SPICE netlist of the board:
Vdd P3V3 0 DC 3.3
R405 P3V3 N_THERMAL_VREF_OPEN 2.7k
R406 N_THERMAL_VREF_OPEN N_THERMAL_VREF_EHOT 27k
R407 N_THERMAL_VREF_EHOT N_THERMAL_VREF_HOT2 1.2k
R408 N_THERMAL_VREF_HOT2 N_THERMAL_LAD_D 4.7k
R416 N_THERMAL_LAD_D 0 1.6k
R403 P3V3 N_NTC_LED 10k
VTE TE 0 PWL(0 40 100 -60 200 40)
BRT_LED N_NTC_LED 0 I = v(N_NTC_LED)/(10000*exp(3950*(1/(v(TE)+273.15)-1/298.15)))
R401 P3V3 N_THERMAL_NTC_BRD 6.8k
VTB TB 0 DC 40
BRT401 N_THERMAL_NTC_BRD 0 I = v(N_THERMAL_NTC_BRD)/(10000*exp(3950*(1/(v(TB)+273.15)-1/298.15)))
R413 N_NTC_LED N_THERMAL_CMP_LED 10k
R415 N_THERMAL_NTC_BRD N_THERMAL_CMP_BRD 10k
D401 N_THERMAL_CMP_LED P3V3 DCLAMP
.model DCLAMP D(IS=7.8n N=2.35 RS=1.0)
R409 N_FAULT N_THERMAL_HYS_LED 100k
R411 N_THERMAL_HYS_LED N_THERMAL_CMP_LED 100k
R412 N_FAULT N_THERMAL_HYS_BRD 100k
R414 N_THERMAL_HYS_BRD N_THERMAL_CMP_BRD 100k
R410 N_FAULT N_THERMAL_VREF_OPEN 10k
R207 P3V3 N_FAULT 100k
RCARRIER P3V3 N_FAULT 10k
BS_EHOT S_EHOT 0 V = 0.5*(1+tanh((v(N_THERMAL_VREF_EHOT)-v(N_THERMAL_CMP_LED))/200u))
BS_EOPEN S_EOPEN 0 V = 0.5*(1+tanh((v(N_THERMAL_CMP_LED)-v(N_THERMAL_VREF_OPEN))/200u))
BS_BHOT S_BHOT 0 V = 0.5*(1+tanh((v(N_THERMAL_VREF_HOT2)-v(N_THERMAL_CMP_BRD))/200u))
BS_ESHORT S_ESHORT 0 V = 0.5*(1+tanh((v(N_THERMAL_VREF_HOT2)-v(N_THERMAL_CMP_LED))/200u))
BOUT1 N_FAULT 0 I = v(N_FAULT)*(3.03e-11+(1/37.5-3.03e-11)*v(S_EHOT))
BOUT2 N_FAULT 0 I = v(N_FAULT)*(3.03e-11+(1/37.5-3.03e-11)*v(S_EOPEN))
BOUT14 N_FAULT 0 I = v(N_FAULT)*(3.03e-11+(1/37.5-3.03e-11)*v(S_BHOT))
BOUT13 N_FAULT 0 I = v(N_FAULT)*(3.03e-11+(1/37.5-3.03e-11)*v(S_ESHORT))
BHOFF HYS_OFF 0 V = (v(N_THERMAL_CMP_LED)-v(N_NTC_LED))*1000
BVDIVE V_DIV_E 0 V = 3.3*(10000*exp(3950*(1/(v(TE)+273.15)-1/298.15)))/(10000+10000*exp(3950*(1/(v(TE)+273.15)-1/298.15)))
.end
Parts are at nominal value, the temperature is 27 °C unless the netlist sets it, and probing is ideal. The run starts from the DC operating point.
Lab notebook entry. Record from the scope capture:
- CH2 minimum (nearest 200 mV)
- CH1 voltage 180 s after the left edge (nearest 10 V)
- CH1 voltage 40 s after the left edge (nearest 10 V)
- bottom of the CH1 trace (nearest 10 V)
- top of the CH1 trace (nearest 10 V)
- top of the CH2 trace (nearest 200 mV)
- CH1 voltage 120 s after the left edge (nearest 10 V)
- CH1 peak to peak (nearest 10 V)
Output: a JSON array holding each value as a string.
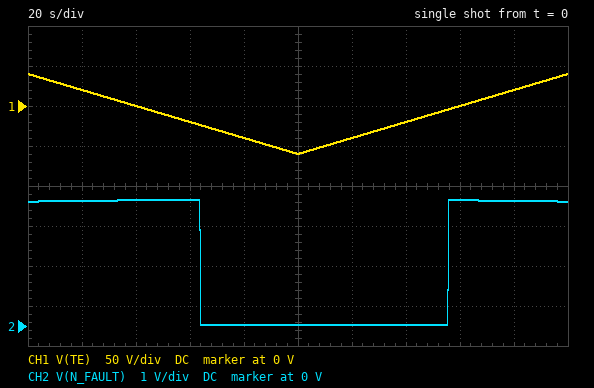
["0 V", "20 V", "0 V", "-60 V", "40 V", "3.2 V", "-40 V", "100 V"]
